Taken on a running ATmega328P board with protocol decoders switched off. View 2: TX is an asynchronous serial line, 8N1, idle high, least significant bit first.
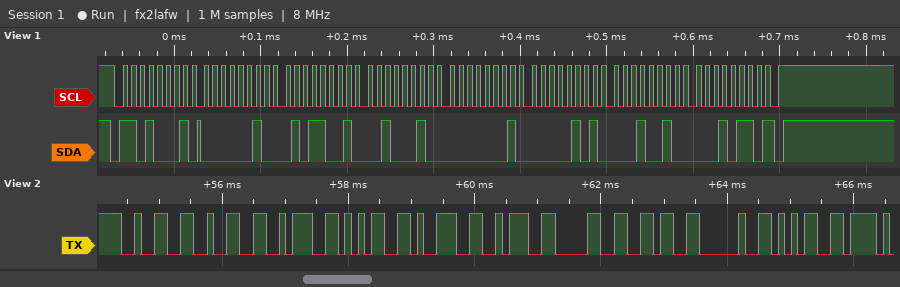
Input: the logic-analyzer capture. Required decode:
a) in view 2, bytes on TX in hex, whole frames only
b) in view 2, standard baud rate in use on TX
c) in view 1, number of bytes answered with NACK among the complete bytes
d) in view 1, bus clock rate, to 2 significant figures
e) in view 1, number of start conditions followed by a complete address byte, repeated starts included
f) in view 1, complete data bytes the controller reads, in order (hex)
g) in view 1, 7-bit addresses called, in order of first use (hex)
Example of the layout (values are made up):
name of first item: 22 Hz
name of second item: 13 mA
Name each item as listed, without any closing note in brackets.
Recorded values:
in view 2, bytes on TX in hex, whole frames only: 32 32 3A 35 39 3A 30 36 20 35
in view 2, standard baud rate in use on TX: 9600 baud
in view 1, number of bytes answered with NACK among the complete bytes: 1
in view 1, bus clock rate, to 2 significant figures: 100 kHz
in view 1, number of start conditions followed by a complete address byte, repeated starts included: 1
in view 1, complete data bytes the controller reads, in order: 02 59 22 01 05 12 16
in view 1, 7-bit addresses called, in order of first use: 0x68
